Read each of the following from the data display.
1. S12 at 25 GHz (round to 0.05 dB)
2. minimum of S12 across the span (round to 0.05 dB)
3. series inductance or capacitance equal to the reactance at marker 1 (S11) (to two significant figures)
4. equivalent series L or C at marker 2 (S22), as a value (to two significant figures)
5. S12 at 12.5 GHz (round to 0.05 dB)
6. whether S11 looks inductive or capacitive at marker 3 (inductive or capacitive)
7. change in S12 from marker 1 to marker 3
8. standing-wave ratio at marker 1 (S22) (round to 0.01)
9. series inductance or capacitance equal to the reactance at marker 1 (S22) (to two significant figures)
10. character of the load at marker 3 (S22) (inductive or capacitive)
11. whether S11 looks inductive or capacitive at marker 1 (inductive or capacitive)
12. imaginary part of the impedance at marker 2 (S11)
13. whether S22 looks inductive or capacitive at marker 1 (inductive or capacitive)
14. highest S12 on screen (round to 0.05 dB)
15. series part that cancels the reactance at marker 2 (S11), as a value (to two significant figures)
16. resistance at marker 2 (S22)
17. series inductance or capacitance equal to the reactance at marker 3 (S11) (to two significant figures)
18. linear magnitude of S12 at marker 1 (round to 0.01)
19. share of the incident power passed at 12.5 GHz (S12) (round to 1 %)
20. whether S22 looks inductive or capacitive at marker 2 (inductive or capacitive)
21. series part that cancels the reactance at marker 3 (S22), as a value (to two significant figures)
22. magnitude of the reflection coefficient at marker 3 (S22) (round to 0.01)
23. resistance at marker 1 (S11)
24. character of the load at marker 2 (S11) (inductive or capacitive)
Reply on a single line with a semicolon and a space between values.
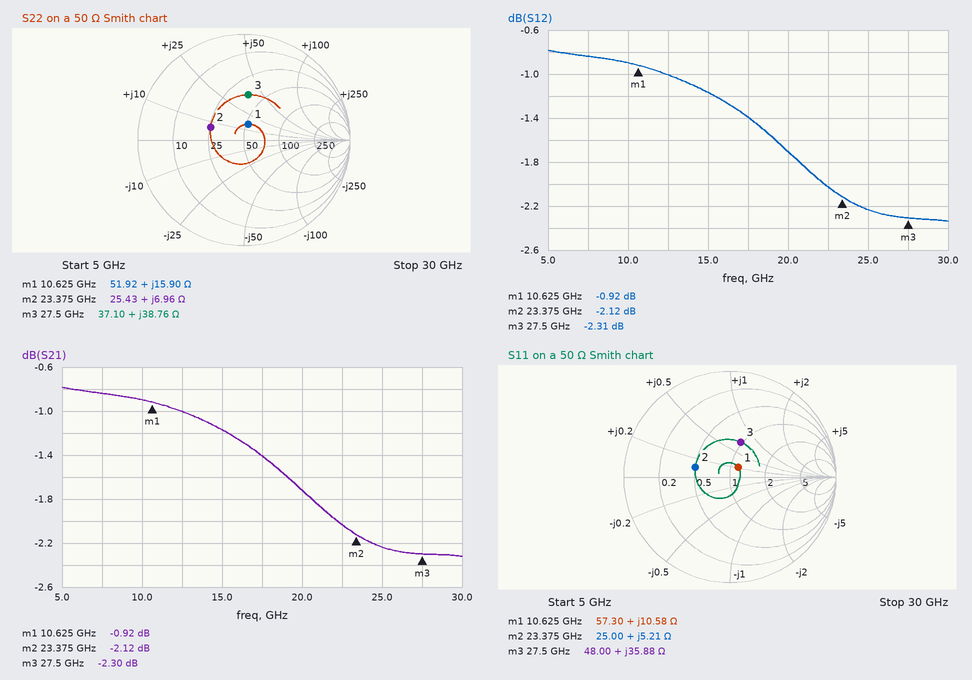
-2.25 dB; -2.35 dB; 160 pH; 47 pH; -1.00 dB; inductive; -1.39 dB; 1.37; 240 pH; inductive; inductive; +5.21 Ω; inductive; -0.80 dB; 1.3 pF; 25.43 Ω; 210 pH; 0.90; 79 %; inductive; 150 fF; 0.43; 57.30 Ω; inductive
